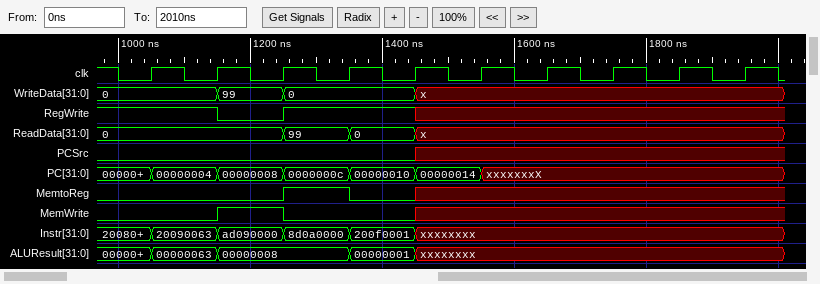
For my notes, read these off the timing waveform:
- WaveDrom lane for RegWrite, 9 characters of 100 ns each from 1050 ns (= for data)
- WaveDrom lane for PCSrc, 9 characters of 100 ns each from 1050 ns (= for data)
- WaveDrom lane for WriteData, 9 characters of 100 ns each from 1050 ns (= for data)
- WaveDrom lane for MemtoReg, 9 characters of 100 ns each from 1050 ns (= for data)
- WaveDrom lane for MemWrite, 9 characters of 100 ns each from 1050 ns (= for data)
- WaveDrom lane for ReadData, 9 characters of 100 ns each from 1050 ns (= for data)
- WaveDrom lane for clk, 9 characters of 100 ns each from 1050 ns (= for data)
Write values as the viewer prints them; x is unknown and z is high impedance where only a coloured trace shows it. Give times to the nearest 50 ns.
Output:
{name: 'RegWrite', wave: '101.x....'}
{name: 'PCSrc', wave: '0...x....'}
{name: 'WriteData', wave: '===.x....', data: '0 99 0'}
{name: 'MemtoReg', wave: '0.10x....'}
{name: 'MemWrite', wave: '010.x....'}
{name: 'ReadData', wave: '=.==x....', data: '0 99 0'}
{name: 'clk', wave: 'p........'}
